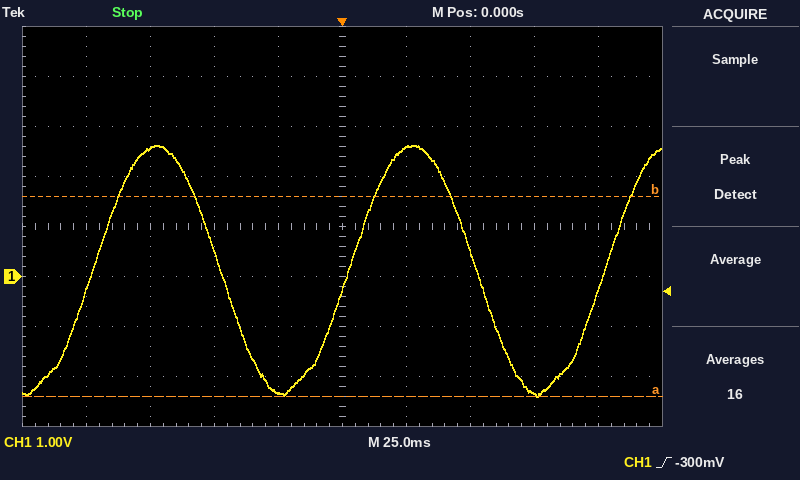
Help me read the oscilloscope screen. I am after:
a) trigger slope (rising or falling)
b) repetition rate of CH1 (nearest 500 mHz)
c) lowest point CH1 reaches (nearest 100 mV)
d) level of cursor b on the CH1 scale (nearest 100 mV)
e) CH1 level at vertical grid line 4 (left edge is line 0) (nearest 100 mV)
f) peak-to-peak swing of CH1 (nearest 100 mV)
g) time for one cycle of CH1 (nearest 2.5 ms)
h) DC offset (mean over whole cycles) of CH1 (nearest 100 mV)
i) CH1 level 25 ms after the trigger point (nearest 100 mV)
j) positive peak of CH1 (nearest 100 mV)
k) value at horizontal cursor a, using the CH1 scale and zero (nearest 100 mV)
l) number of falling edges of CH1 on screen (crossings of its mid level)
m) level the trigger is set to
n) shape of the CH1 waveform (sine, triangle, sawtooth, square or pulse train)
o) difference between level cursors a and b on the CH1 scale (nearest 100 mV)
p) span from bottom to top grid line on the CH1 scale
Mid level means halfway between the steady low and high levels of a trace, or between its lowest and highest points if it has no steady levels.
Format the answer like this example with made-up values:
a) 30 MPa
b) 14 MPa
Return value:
a) rising
b) 10.0 Hz
c) -2.4 V
d) 1.6 V
e) -2.3 V
f) 5.0 V
g) 100.0 ms
h) 100 mV
i) 2.6 V
j) 2.6 V
k) -2.4 V
l) 2
m) -300 mV
n) sine
o) 4.0 V
p) 8 V
